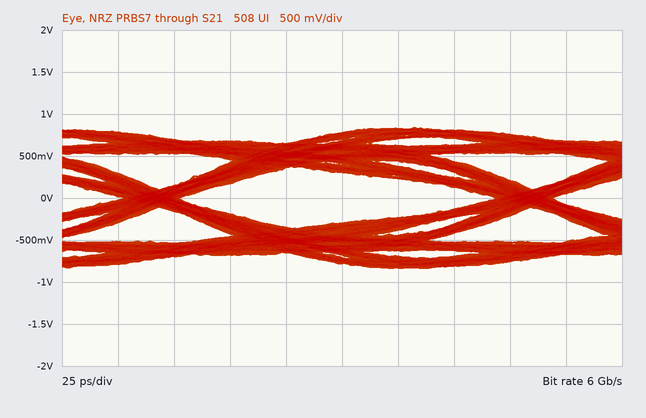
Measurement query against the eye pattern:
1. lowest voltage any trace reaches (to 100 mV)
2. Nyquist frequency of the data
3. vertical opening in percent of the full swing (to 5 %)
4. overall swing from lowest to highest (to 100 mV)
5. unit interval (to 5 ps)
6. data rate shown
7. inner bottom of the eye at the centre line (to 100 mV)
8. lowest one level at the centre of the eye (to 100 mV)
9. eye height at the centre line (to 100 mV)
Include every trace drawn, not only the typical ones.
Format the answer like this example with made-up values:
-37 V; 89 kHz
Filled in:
-800 mV; 3 GHz; 35 %; 1.7 V; 165 ps; 6 Gb/s; -300 mV; 300 mV; 600 mV
